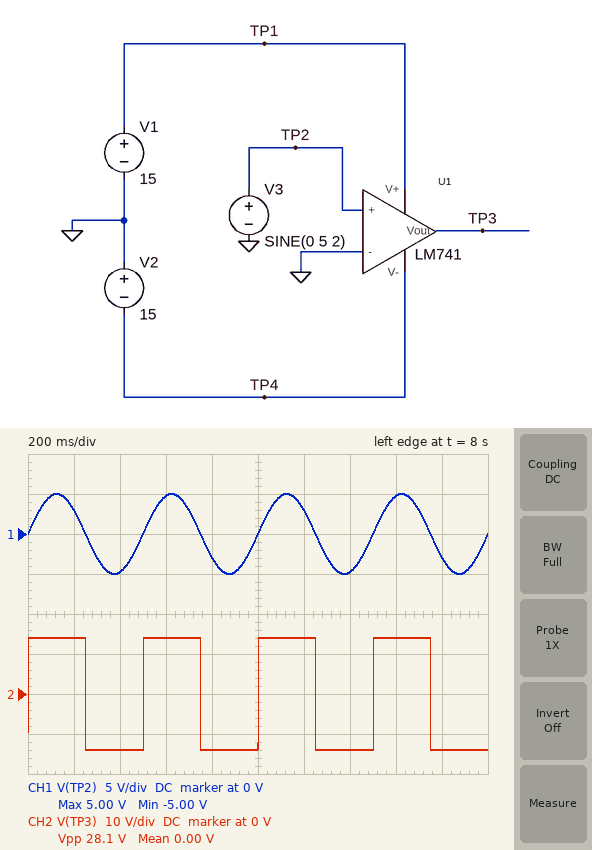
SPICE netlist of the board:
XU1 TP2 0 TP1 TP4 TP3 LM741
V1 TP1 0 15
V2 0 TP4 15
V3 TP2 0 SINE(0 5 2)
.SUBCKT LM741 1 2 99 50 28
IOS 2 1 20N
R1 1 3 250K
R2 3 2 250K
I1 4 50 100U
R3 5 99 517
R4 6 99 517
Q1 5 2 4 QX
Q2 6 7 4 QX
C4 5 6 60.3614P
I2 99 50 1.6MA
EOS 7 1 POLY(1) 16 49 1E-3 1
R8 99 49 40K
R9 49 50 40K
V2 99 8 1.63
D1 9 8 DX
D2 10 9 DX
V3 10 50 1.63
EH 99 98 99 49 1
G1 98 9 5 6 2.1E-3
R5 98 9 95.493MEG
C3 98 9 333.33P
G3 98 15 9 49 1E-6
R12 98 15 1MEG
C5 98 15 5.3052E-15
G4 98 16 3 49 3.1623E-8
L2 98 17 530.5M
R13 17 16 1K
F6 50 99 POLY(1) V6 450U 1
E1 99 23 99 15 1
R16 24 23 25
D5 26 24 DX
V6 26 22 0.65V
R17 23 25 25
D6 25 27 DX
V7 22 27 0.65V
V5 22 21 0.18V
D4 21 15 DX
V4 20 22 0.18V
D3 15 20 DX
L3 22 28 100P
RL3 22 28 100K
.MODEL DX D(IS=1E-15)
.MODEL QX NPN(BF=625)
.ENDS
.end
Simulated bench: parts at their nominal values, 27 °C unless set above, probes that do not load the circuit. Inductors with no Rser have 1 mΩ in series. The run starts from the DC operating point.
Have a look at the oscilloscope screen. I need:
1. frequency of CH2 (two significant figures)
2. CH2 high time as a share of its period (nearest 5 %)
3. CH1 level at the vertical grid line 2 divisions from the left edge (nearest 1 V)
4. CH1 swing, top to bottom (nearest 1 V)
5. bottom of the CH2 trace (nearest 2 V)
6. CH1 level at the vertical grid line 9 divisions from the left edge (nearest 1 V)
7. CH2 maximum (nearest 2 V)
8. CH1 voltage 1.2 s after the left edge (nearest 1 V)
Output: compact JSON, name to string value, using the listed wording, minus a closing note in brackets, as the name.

{"frequency of CH2": "2.0 Hz", "CH2 high time as a share of its period": "50 %", "CH1 level at the vertical grid line 2 divisions from the left edge": "-5 V", "CH1 swing, top to bottom": "10 V", "bottom of the CH2 trace": "-14 V", "CH1 level at the vertical grid line 9 divisions from the left edge": "-3 V", "CH2 maximum": "14 V", "CH1 voltage 1.2 s after the left edge": "3 V"}
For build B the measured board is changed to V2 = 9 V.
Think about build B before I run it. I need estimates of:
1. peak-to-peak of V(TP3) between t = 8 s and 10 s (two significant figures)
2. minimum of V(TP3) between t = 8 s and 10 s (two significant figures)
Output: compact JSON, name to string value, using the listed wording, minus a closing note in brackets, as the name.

{"peak-to-peak of V(TP3) between t = 8 s and 10 s": "22 V", "minimum of V(TP3) between t = 8 s and 10 s": "-8.0 V"}
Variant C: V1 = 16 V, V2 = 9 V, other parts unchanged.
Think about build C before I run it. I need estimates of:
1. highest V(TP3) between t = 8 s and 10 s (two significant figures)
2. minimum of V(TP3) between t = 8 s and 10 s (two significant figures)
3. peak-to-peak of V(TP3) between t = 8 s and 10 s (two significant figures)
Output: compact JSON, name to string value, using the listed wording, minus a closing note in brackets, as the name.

{"highest V(TP3) between t = 8 s and 10 s": "15 V", "minimum of V(TP3) between t = 8 s and 10 s": "-8.0 V", "peak-to-peak of V(TP3) between t = 8 s and 10 s": "23 V"}
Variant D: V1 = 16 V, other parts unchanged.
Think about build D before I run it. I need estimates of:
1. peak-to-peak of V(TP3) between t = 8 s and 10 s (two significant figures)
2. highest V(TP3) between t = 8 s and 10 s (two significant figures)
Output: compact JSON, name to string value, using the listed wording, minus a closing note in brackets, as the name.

{"peak-to-peak of V(TP3) between t = 8 s and 10 s": "29 V", "highest V(TP3) between t = 8 s and 10 s": "15 V"}
